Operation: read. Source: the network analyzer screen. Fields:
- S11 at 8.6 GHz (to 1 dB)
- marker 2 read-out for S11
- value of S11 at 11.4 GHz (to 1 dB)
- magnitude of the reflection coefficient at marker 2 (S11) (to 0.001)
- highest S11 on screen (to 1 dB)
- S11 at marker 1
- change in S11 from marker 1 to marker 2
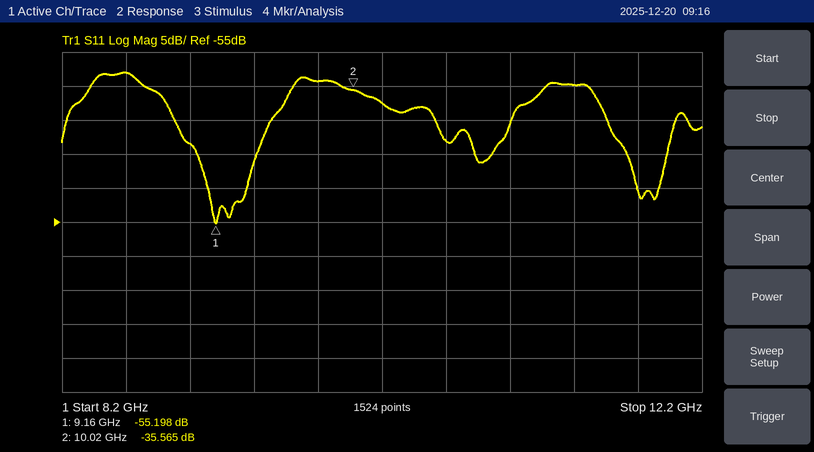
-33 dB
-35.565 dB
-35 dB
0.017
-33 dB
-55.198 dB
19.633 dB
